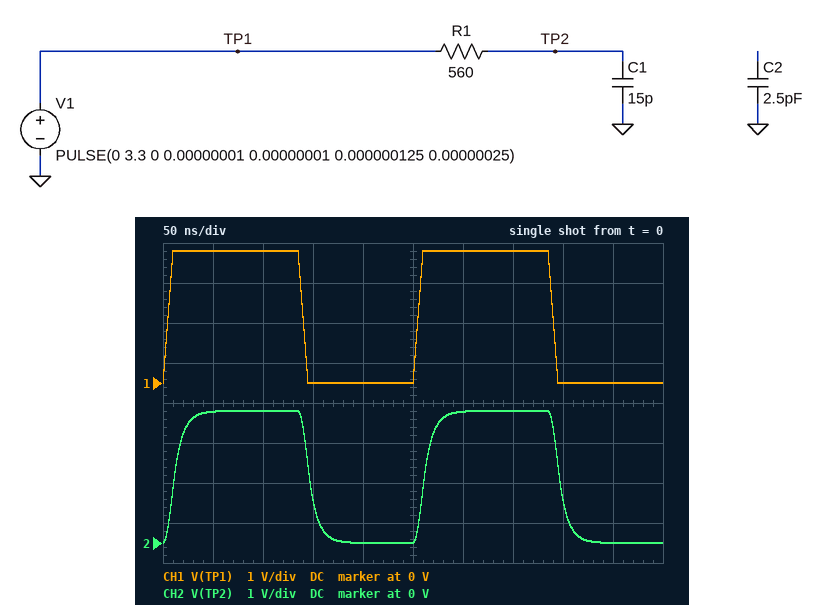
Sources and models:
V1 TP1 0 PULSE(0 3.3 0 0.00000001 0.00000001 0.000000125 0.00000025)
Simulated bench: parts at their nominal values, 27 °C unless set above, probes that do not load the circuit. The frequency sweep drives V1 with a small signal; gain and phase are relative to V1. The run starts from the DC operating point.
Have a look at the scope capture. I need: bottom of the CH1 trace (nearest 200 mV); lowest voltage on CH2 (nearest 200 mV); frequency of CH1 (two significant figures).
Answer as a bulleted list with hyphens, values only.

- 0 V
- 0 V
- 4.0 MHz
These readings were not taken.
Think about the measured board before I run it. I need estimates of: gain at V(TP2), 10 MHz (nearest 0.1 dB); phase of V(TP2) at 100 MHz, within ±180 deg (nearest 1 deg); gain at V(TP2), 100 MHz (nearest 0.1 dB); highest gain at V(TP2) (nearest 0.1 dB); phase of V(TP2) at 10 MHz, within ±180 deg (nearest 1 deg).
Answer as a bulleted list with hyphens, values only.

- -1.1 dB
- -79 deg
- -14.6 dB
- 0 dB
- -28 deg
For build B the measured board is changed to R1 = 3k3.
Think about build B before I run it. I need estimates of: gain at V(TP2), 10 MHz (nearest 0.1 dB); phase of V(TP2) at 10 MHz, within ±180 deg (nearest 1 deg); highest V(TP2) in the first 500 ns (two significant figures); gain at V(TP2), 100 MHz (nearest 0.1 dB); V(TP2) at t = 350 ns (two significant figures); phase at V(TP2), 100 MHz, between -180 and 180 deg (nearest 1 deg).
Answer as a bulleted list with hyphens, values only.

- -10.3 dB
- -72 deg
- 3.1 V
- -29.9 dB
- 2.9 V
- -88 deg
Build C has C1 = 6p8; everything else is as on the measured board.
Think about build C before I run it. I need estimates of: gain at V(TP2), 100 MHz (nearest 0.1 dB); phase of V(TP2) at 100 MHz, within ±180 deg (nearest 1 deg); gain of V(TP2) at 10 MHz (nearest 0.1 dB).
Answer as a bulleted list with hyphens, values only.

- -8.3 dB
- -67 deg
- -0.2 dB
